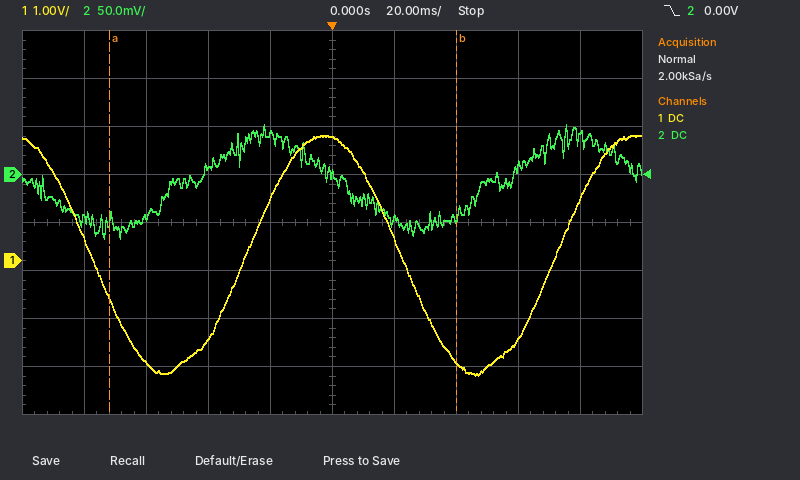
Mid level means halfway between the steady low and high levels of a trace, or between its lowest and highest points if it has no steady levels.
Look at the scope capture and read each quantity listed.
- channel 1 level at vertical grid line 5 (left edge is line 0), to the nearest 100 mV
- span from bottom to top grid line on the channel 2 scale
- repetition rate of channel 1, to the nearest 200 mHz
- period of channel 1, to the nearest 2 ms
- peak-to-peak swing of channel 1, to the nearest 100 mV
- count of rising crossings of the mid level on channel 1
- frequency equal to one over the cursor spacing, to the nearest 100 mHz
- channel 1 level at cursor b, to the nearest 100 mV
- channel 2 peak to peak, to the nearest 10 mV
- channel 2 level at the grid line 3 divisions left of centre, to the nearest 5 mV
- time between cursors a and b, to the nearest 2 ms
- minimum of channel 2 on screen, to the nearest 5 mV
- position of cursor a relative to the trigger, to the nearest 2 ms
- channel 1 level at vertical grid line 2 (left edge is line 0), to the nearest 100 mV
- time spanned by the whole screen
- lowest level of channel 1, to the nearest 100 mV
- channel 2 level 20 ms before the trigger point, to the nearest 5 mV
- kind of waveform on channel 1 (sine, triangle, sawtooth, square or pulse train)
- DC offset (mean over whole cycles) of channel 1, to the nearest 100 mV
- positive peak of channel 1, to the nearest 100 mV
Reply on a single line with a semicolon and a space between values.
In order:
2.6 V; 400 mV; 10.0 Hz; 100 ms; 5.0 V; 2; 8.9 Hz; -2.1 V; 120 mV; -45 mV; 112 ms; -65 mV; -72 ms; -2.1 V; 200 ms; -2.4 V; 45 mV; sine; 100 mV; 2.6 V
